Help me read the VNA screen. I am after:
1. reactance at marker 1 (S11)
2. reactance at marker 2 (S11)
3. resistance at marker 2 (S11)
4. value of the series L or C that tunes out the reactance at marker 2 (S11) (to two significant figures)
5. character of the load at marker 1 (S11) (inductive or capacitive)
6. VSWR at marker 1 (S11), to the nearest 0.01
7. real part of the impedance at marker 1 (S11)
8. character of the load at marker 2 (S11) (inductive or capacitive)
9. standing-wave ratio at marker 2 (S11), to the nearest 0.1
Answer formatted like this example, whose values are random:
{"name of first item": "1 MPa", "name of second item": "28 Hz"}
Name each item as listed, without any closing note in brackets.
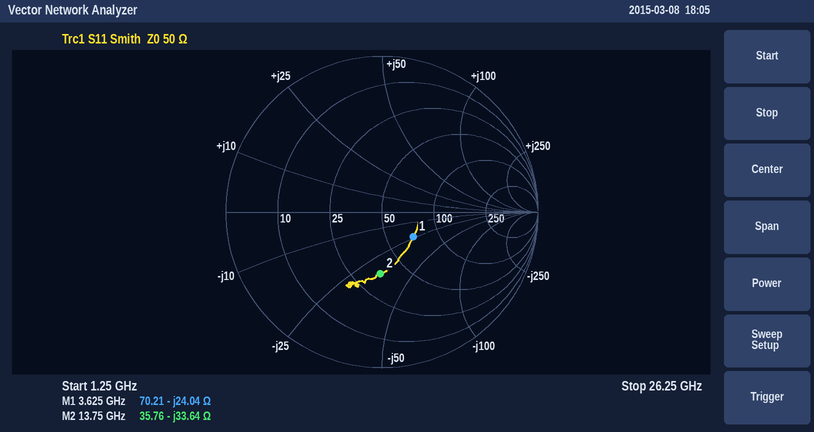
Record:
{"reactance at marker 1": "-24.04 Ω", "reactance at marker 2": "-33.64 Ω", "resistance at marker 2": "35.76 Ω", "value of the series L or C that tunes out the reactance at marker 2 (S11)": "390 pH", "character of the load at marker 1 (S11)": "capacitive", "VSWR at marker 1 (S11), to the nearest 0.01": "1.69", "real part of the impedance at marker 1": "70.21 Ω", "character of the load at marker 2 (S11)": "capacitive", "standing-wave ratio at marker 2 (S11), to the nearest 0.1": "2.3"}
